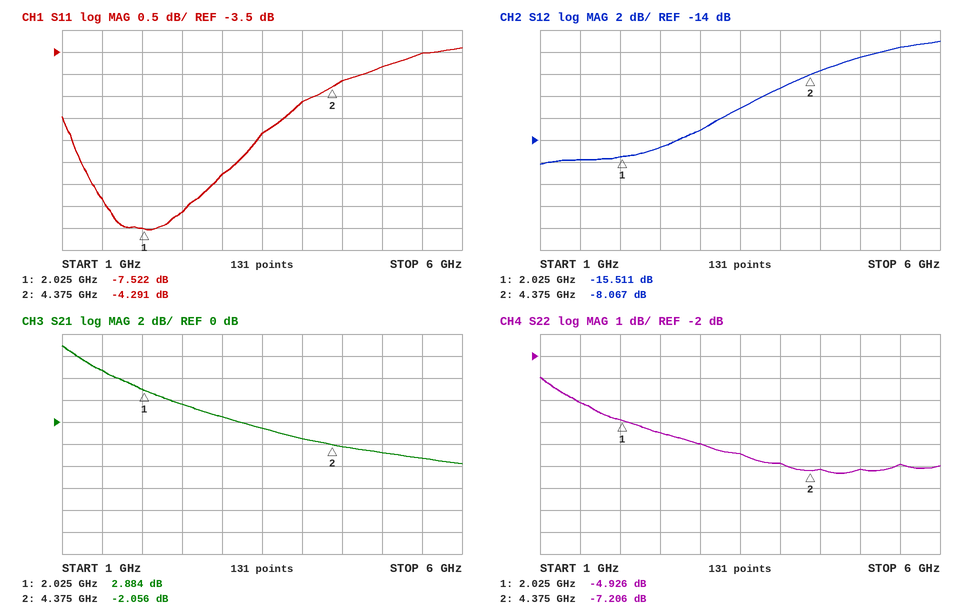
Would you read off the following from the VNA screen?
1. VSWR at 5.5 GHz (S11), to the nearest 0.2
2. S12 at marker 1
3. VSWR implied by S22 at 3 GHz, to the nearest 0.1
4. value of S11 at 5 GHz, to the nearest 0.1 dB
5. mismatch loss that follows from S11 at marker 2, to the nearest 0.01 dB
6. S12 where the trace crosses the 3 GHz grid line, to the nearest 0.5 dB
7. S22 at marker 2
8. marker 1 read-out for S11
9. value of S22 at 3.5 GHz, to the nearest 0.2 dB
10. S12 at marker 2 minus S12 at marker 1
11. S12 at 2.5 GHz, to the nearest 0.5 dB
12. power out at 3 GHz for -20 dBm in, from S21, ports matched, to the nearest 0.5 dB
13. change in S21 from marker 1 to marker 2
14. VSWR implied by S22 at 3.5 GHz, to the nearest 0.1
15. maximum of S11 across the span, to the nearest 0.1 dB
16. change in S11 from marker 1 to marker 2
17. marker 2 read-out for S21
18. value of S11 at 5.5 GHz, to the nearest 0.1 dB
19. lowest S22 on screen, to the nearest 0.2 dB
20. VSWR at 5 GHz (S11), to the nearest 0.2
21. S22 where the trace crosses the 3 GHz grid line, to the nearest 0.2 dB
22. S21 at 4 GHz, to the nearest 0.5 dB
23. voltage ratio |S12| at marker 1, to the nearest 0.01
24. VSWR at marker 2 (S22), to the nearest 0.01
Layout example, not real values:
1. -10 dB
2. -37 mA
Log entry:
1. 5.0
2. -15.511 dB
3. 3.0
4. -3.8 dB
5. 2.02 dB
6. -13.0 dB
7. -7.206 dB
8. -7.522 dB
9. -6.4 dB
10. 7.444 dB
11. -14.5 dB
12. -19.5 dBm
13. -4.940 dB
14. 2.8
15. -3.4 dB
16. 3.231 dB
17. -2.056 dB
18. -3.5 dB
19. -7.4 dB
20. 4.6
21. -6.0 dB
22. -1.5 dB
23. 0.17
24. 2.55
